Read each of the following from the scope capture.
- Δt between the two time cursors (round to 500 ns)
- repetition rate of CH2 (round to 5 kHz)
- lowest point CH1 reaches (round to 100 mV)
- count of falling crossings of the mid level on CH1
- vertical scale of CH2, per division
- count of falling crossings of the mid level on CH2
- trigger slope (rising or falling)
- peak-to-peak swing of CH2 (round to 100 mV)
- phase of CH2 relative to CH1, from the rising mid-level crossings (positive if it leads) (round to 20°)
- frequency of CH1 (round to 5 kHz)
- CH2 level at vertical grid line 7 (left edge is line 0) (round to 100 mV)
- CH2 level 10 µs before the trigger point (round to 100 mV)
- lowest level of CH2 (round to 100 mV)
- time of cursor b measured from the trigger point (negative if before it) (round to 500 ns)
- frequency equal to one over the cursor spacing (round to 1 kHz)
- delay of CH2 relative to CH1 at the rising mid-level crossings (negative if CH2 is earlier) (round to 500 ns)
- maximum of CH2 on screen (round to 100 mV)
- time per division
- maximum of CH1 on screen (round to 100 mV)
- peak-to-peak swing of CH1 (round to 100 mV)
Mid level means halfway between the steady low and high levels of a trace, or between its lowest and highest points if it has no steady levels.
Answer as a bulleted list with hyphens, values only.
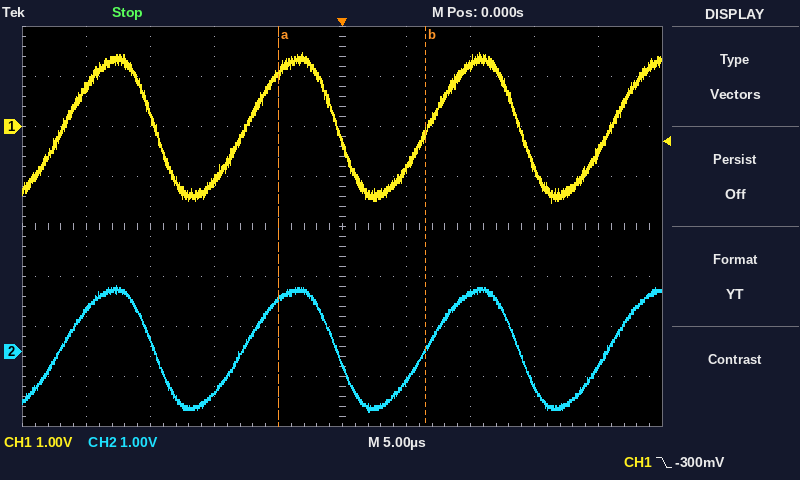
- 11.5 µs
- 70 kHz
- -1.5 V
- 3
- 1 V
- 3
- falling
- 2.5 V
- 0°
- 70 kHz
- 1.2 V
- -800 mV
- -1.2 V
- +6.5 µs
- 87 kHz
- 0.0 µs
- 1.3 V
- 5 µs
- 1.5 V
- 3.0 V
